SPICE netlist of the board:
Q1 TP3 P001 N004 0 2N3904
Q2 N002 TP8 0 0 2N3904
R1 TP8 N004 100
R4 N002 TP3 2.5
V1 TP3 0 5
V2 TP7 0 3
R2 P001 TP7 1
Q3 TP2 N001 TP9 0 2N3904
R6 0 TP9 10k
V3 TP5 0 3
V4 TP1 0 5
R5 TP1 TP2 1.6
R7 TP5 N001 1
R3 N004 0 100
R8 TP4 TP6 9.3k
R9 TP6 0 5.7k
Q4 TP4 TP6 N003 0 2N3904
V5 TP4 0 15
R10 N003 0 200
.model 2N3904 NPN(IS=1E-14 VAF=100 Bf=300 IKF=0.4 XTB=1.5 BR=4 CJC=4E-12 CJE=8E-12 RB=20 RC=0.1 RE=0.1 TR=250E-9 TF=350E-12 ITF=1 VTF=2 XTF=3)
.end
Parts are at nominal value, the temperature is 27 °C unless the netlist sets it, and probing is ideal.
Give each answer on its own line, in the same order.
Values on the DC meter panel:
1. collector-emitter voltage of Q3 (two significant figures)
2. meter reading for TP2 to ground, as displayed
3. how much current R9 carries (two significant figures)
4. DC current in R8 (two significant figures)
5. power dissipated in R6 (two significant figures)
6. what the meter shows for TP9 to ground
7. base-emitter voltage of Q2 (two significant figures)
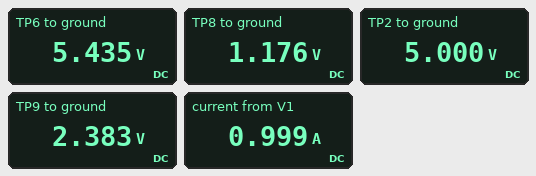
2.6 V
5.000 V
950 µA
1.0 mA
570 µW
2.383 V
1.2 V
